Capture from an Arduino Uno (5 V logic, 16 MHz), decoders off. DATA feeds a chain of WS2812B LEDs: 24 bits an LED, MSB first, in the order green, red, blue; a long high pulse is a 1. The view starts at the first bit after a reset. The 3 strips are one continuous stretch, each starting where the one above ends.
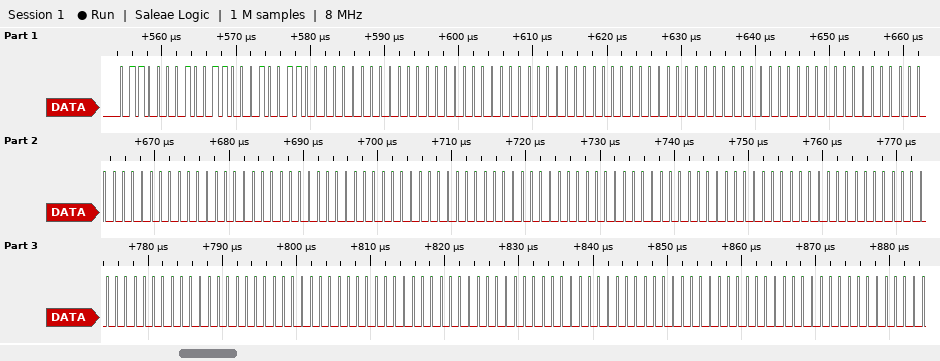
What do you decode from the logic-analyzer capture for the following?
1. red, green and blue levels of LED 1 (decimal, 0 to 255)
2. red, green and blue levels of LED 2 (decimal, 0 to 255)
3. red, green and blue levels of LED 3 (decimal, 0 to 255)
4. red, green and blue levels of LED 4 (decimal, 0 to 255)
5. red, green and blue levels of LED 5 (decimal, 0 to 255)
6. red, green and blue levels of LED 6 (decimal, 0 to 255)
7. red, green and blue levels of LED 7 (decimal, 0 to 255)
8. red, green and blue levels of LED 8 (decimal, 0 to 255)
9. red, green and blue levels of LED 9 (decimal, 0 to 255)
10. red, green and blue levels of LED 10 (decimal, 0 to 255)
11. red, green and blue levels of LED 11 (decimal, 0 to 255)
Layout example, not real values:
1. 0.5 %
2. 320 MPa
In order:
1. 49, 97, 48
2. 0, 0, 0
3. 0, 0, 0
4. 0, 0, 0
5. 0, 0, 0
6. 0, 0, 0
7. 0, 0, 0
8. 0, 0, 0
9. 0, 0, 0
10. 0, 0, 0
11. 0, 0, 0
